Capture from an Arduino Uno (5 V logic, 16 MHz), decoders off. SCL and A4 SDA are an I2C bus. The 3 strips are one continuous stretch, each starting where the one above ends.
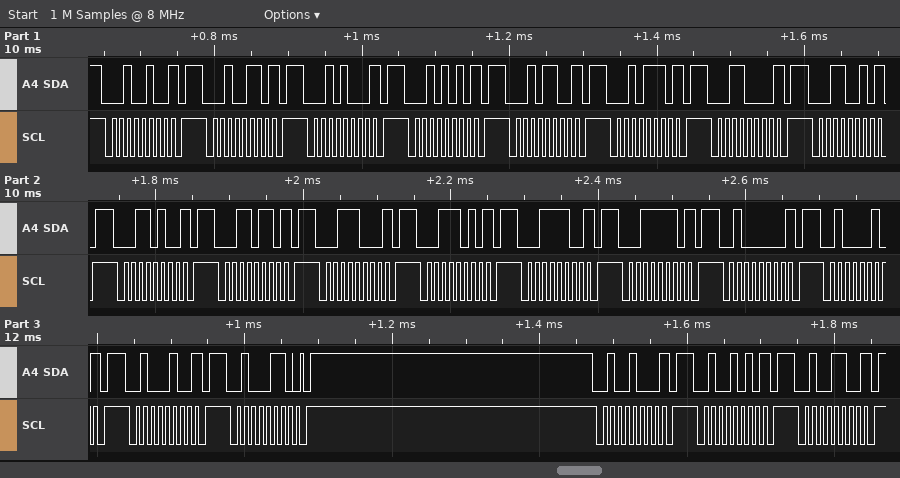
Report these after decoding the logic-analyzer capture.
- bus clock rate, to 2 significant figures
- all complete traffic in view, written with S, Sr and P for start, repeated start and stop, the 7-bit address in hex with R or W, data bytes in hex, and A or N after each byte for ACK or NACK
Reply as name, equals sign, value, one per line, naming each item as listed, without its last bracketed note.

bus clock rate, to 2 significant figures = 100 kHz
all complete traffic in view, written with S, Sr and P for start, repeated start and stop, the 7-bit address in hex with R or W, data bytes in hex, and A or N after each byte for ACK or NACK = S 12W N P S 13W N P S 14W N P S 15W N P S 16W N P S 17W N P S 18W N P S 19W N P S 1AW N P S 1BW N P S 1CW N P S 1DW N P S 1EW N P S 1FW N P S 20W N P S 21W N P S 22W N P S 23W A P S 24W N P S 25W N P S 26W N P
